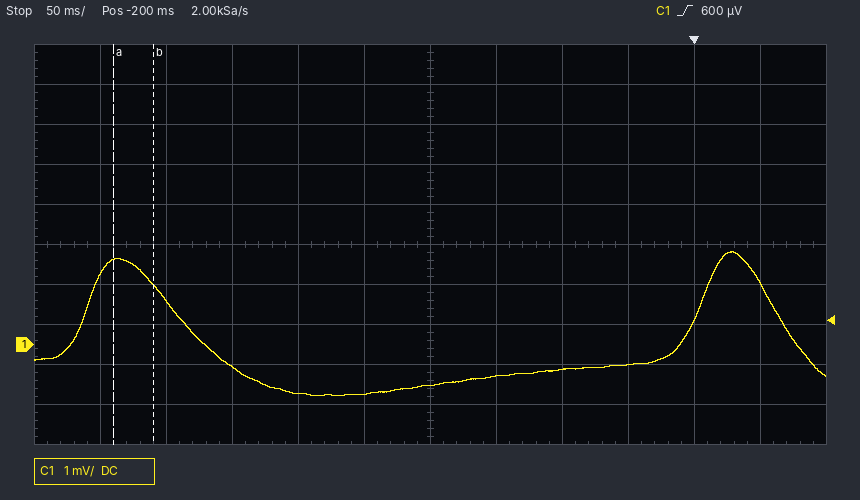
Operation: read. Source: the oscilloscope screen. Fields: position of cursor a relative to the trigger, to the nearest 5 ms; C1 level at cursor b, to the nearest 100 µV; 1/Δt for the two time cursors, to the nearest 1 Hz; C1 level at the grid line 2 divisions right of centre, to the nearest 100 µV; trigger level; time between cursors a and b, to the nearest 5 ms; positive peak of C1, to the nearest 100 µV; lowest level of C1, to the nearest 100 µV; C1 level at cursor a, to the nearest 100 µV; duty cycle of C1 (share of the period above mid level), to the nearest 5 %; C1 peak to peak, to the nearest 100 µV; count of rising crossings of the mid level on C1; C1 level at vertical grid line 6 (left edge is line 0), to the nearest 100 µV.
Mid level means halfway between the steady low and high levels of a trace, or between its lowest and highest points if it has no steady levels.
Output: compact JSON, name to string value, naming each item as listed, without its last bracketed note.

{"position of cursor a relative to the trigger, to the nearest 5 ms": "-440 ms", "C1 level at cursor b, to the nearest 100 µV": "1.5 mV", "1/Δt for the two time cursors, to the nearest 1 Hz": "33 Hz", "C1 level at the grid line 2 divisions right of centre, to the nearest 100 µV": "-600 µV", "trigger level": "600 µV", "time between cursors a and b, to the nearest 5 ms": "30 ms", "positive peak of C1, to the nearest 100 µV": "2.3 mV", "lowest level of C1, to the nearest 100 µV": "-1.3 mV", "C1 level at cursor a, to the nearest 100 µV": "2.1 mV", "duty cycle of C1 (share of the period above mid level), to the nearest 5 %": "15 %", "C1 peak to peak, to the nearest 100 µV": "3.6 mV", "count of rising crossings of the mid level on C1": "2", "C1 level at vertical grid line 6 (left edge is line 0), to the nearest 100 µV": "-1.0 mV"}
